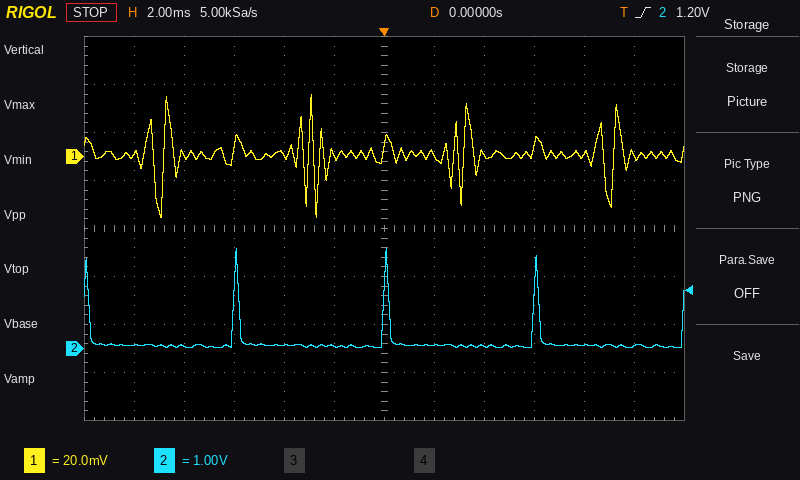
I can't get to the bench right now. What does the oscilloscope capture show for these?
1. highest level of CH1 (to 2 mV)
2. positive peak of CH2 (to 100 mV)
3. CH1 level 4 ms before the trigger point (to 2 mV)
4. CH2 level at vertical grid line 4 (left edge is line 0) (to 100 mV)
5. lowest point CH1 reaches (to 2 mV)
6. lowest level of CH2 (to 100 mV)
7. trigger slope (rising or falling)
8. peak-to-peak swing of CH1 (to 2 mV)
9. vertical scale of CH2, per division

26 mV
2.1 V
0 mV
100 mV
-26 mV
0.0 V
rising
52 mV
1 V
